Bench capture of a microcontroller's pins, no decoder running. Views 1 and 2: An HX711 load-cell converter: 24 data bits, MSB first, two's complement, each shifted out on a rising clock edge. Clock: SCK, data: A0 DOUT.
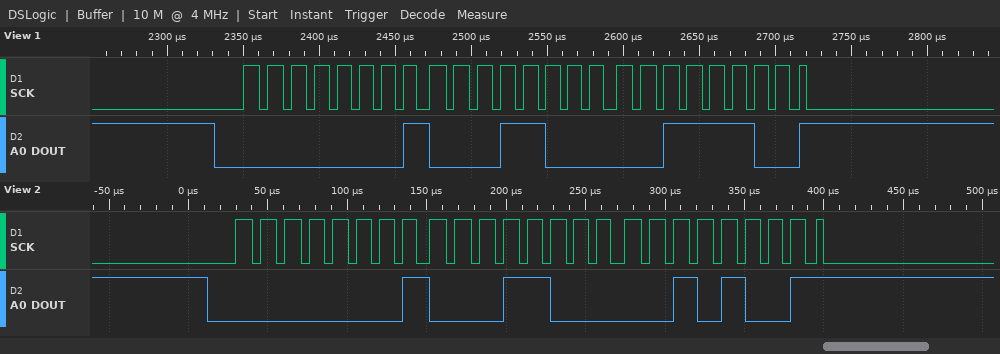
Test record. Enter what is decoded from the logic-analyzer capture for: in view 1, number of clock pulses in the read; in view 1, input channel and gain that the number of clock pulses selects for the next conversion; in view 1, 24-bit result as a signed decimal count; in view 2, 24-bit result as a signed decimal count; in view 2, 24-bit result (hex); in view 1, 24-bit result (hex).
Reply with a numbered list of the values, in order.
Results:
1. 25
2. channel A, gain 128
3. 71740
4. 71721
5. 0x011829
6. 0x01183C
